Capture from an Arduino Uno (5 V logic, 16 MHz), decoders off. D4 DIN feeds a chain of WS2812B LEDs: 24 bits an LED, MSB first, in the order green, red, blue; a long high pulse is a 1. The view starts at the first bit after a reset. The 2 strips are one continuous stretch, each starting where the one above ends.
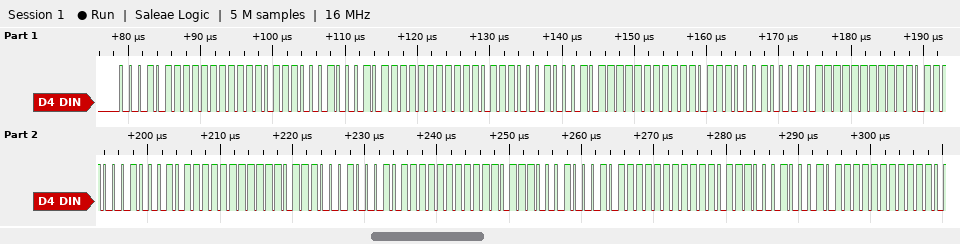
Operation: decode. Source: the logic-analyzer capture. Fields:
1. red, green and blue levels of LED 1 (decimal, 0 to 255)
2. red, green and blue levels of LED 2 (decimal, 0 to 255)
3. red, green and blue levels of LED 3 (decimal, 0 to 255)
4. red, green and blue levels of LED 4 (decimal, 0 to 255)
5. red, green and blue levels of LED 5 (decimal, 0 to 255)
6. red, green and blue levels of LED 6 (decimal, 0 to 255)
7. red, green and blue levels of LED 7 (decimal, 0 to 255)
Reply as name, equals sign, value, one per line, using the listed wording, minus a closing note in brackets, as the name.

red, green and blue levels of LED 1 = 255, 23, 113
red, green and blue levels of LED 2 = 255, 23, 113
red, green and blue levels of LED 3 = 255, 23, 113
red, green and blue levels of LED 4 = 255, 23, 113
red, green and blue levels of LED 5 = 255, 23, 113
red, green and blue levels of LED 6 = 255, 23, 113
red, green and blue levels of LED 7 = 255, 23, 113
